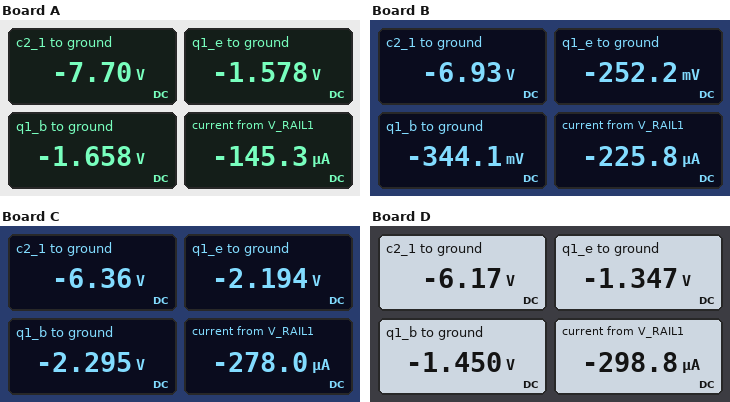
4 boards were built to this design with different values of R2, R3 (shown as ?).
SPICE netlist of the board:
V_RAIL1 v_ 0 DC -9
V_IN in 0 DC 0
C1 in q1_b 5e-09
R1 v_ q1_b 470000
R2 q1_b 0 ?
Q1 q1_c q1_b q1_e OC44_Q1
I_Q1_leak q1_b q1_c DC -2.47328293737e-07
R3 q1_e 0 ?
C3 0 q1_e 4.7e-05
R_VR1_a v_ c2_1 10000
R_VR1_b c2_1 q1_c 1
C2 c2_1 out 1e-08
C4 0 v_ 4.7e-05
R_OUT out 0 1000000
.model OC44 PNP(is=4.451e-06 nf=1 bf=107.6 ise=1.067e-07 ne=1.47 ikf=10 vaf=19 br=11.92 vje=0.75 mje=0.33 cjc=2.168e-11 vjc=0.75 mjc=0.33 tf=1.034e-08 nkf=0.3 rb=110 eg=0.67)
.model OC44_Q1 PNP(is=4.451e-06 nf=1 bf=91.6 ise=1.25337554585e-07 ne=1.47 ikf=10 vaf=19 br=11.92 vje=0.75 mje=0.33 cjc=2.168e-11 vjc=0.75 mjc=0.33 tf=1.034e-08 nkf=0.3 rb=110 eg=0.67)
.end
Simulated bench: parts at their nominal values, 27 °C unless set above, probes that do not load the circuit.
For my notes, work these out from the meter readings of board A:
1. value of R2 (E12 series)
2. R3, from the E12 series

120 kΩ
12 kΩ
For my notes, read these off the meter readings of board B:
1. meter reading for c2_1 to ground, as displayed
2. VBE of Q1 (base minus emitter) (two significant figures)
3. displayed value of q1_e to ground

-6.93 V
-92 mV
-252.2 mV
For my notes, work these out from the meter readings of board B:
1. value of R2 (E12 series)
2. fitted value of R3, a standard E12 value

22 kΩ
1.2 kΩ
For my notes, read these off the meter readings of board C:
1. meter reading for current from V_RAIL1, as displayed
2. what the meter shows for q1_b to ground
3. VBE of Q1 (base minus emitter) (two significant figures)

-278.0 µA
-2.295 V
-100 mV
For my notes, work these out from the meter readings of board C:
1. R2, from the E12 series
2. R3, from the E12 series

220 kΩ
8.2 kΩ
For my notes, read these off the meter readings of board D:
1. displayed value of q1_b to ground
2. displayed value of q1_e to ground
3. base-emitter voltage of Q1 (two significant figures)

-1.450 V
-1.347 V
-100 mV
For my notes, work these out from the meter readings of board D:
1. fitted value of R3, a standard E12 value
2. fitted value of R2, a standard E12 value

4.7 kΩ
120 kΩ
